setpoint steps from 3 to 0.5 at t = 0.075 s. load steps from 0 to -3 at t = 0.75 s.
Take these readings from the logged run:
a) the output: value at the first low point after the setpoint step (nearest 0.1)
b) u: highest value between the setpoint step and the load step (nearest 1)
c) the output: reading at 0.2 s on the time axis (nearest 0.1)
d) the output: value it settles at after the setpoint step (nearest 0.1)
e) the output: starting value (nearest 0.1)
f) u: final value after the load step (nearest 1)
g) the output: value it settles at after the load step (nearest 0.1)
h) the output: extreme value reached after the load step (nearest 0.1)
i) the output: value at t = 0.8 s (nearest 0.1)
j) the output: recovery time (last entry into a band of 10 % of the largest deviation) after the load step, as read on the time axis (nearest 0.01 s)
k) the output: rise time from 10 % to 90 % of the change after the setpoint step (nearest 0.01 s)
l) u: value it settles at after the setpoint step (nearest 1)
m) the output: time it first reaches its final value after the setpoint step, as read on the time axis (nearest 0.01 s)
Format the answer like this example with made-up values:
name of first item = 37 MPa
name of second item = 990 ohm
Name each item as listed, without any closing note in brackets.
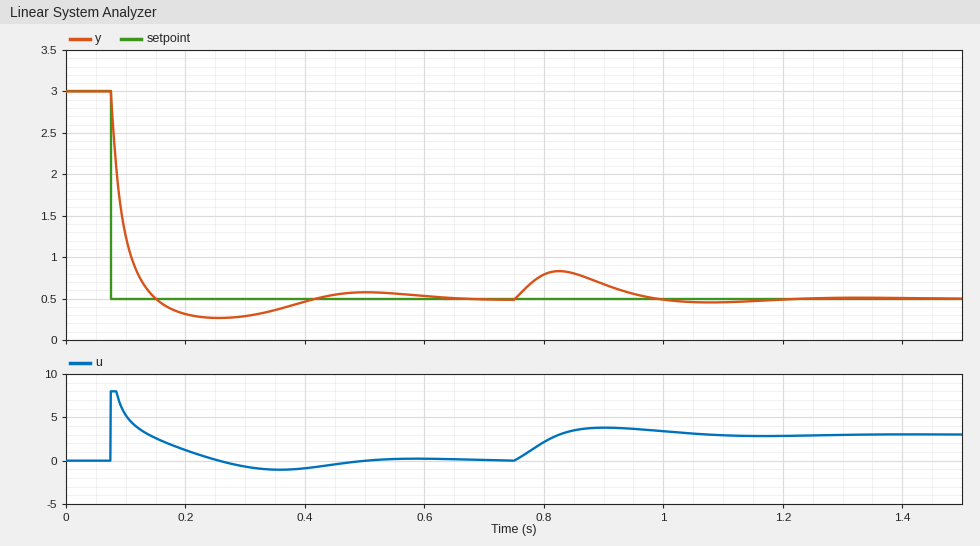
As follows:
the output: value at the first low point after the setpoint step = 0.3
u: highest value between the setpoint step and the load step = 8
the output: reading at 0.2 s on the time axis = 0.3
the output: value it settles at after the setpoint step = 0.5
the output: starting value = 3.0
u: final value after the load step = 3
the output: value it settles at after the load step = 0.5
the output: extreme value reached after the load step = 0.8
the output: value at t = 0.8 s = 0.8
the output: recovery time (last entry into a band of 10 % of the largest deviation) after the load step, as read on the time axis = 1.14 s
the output: rise time from 10 % to 90 % of the change after the setpoint step = 0.05 s
u: value it settles at after the setpoint step = 0
the output: time it first reaches its final value after the setpoint step, as read on the time axis = 0.15 s
